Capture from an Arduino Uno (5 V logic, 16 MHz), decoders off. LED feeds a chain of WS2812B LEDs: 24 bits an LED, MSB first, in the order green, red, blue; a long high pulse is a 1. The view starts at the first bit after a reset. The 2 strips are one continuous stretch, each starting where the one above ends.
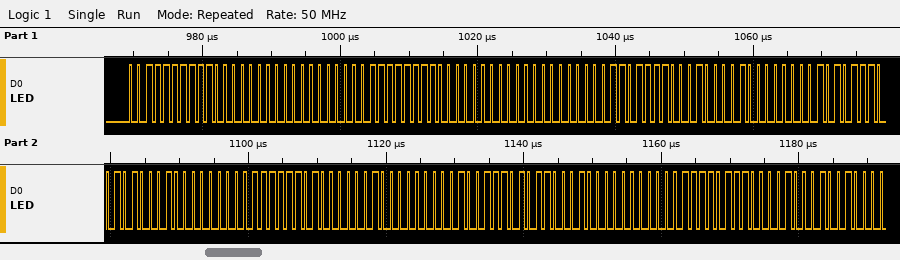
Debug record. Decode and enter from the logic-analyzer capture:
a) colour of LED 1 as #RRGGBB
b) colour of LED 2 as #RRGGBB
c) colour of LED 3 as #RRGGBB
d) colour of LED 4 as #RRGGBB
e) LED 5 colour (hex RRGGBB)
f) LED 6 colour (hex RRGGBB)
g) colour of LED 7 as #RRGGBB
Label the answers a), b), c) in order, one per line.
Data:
a) #C03F00
b) #F00F00
c) #DE0021
d) #AE0051
e) #7E0081
f) #4E00B1
g) #1E00E1
